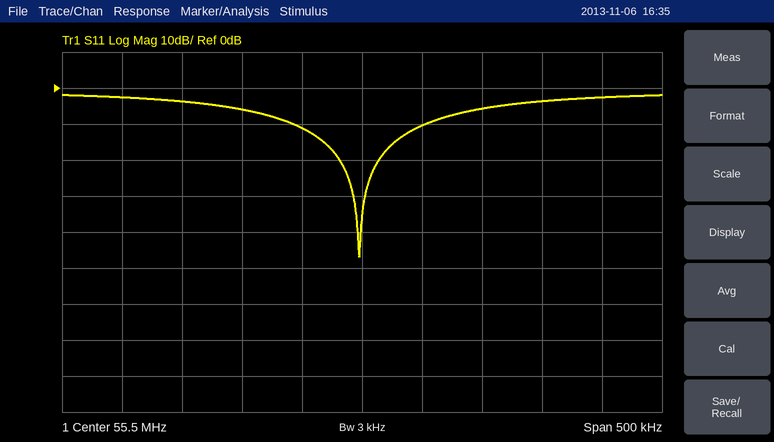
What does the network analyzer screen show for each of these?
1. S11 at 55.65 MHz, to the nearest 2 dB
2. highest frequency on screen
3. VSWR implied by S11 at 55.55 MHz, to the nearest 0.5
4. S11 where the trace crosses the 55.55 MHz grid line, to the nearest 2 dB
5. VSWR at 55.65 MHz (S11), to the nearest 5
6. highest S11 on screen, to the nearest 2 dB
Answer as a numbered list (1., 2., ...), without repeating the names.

1. -4 dB
2. 55.75 MHz
3. 2.0
4. -10 dB
5. 5
6. -2 dB
